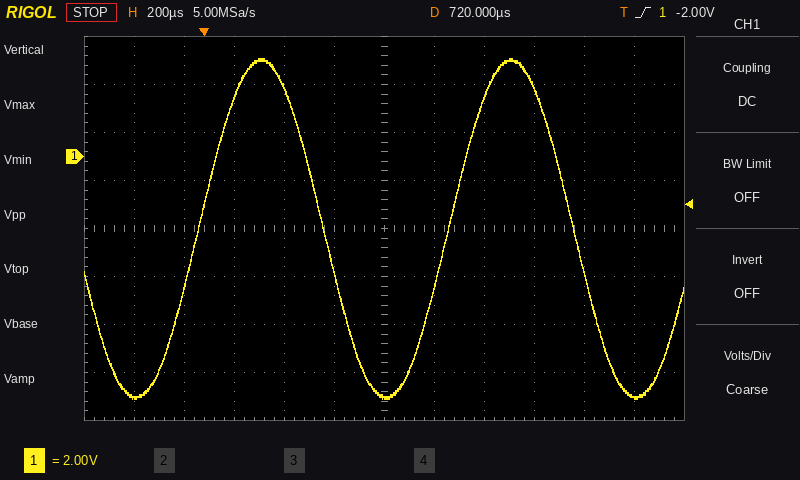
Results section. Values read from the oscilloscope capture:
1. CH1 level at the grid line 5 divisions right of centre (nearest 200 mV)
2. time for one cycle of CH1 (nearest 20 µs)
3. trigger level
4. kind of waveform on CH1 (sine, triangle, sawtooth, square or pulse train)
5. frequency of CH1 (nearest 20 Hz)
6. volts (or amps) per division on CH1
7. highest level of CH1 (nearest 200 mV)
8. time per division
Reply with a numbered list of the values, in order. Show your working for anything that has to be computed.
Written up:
1. -10.0 V
2. 1.00 ms
3. -2.00 V
4. sine
5. 1 / 1.00 ms ≈ 1.00 kHz
6. 2 V
7. 4.0 V
8. 200 µs
